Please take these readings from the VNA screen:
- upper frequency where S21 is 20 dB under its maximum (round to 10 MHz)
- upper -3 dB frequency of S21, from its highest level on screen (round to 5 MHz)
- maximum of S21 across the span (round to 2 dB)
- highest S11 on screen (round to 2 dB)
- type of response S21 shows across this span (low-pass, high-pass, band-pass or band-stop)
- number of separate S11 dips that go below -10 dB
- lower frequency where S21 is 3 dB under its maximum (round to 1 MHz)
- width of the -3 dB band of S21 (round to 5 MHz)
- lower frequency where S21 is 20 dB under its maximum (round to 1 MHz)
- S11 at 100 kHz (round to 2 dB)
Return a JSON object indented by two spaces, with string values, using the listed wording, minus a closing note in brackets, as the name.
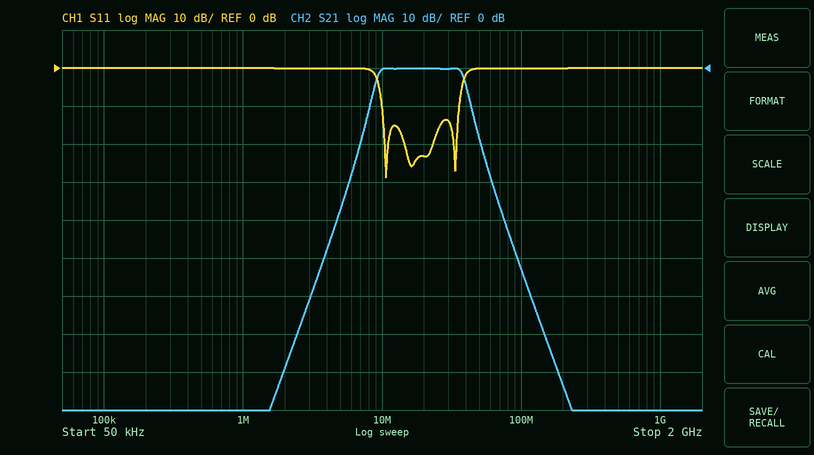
{
  "upper frequency where S21 is 20 dB under its maximum": "50 MHz",
  "upper -3 dB frequency of S21, from its highest level on screen": "40 MHz",
  "maximum of S21 across the span": "0 dB",
  "highest S11 on screen": "0 dB",
  "type of response S21 shows across this span": "band-pass",
  "number of separate S11 dips that go below -10 dB": "3",
  "lower frequency where S21 is 3 dB under its maximum": "9 MHz",
  "width of the -3 dB band of S21": "30 MHz",
  "lower frequency where S21 is 20 dB under its maximum": "7 MHz",
  "S11 at 100 kHz": "0 dB"
}
